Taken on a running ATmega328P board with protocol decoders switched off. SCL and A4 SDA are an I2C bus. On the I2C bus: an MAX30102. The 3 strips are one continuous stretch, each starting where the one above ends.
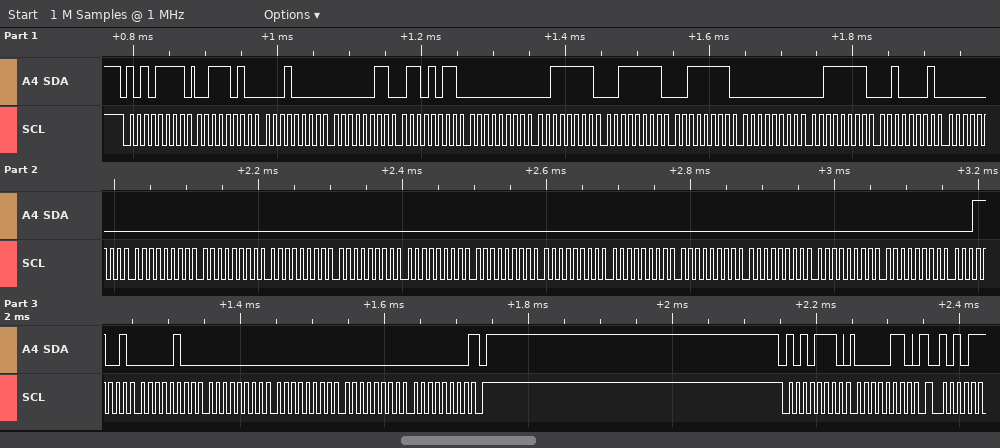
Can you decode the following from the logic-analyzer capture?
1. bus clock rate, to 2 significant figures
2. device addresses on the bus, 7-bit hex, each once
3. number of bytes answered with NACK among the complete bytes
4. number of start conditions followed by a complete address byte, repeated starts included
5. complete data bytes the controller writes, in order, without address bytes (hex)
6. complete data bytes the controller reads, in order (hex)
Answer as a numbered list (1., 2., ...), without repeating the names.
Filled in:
1. 100 kHz
2. 0x57
3. 1
4. 2
5. 06
6. 3A 10 03 6B 00 3F 3F 3F 00 3F 21 00 00 00 00 00 00 00 00 00 00 00 00 00 19 04 00 00 00 00
